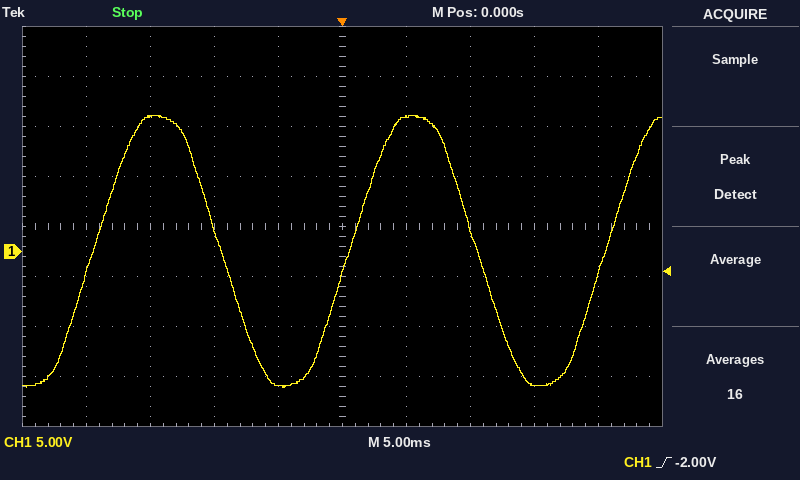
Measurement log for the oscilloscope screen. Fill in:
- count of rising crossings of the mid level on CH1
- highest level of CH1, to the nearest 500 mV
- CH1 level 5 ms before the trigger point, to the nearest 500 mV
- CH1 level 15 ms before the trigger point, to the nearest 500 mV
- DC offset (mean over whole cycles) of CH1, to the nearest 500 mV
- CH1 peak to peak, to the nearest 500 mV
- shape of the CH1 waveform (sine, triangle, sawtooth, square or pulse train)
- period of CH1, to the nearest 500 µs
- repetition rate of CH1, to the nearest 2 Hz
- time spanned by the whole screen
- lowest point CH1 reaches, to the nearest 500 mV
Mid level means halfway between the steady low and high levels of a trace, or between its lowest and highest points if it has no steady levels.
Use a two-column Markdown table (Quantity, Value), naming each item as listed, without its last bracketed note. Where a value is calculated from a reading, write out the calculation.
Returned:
| Quantity | Value |
|---|---|
| count of rising crossings of the mid level on CH1 | 3 |
| highest level of CH1, to the nearest 500 mV | 13.5 V |
| CH1 level 5 ms before the trigger point, to the nearest 500 mV | -13.5 V |
| CH1 level 15 ms before the trigger point, to the nearest 500 mV | 13.5 V |
| DC offset (mean over whole cycles) of CH1, to the nearest 500 mV | (13.5 V + (-13.5 V)) / 2 ≈ 0.0 V |
| CH1 peak to peak, to the nearest 500 mV | 13.5 V − (-13.5 V) = 27.0 V |
| shape of the CH1 waveform | sine |
| period of CH1, to the nearest 500 µs | 20.0 ms |
| repetition rate of CH1, to the nearest 2 Hz | 1 / 20.0 ms ≈ 50 Hz |
| time spanned by the whole screen | 50 ms |
| lowest point CH1 reaches, to the nearest 500 mV | -13.5 V |
